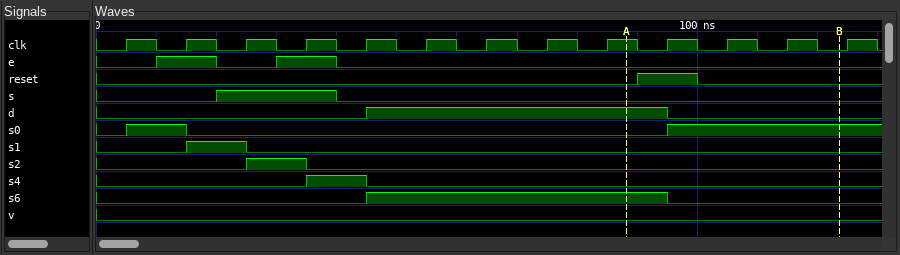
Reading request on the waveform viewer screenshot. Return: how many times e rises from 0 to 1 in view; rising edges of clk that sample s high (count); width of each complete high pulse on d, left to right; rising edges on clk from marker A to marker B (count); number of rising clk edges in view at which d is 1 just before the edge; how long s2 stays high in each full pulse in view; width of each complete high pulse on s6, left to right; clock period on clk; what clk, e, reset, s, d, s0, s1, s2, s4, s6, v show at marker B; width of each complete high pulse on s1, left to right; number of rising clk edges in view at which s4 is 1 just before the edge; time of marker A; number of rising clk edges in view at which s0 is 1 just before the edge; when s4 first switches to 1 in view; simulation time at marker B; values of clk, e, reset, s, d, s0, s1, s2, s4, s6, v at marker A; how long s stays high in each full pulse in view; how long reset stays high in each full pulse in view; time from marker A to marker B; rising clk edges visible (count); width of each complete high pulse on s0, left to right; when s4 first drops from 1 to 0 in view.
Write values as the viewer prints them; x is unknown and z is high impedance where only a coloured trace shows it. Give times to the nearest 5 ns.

2
2
50 ns
3
5
10 ns
50 ns
10 ns
clk=0, e=0, reset=0, s=0, d=0, s0=1, s1=0, s2=0, s4=0, s6=0, v=0
10 ns
1
90 ns
4
35 ns
125 ns
clk=1, e=0, reset=0, s=0, d=1, s0=0, s1=0, s2=0, s4=0, s6=1, v=0
20 ns
10 ns
35 ns
13
10 ns
45 ns
